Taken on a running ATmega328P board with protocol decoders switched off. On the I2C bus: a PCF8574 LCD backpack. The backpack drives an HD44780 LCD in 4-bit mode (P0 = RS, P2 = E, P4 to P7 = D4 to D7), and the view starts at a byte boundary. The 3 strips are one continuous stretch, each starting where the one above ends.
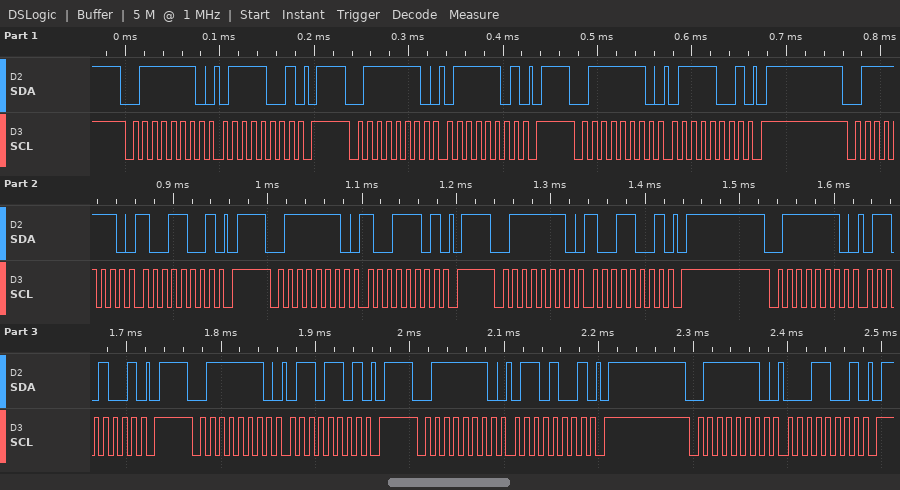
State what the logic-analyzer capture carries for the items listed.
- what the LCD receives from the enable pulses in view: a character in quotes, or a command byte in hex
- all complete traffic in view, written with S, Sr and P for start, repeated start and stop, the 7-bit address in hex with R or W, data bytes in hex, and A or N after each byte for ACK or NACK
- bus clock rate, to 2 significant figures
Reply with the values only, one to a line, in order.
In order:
'y'
S 3FW A 79 A P S 3FW A 7D A P S 3FW A 79 A P S 3FW A 99 A P S 3FW A 9D A P S 3FW A 99 A P S 3FW A 69 A P S 3FW A 6D A P S 3FW A 69 A P S 3FW A 19 A P
100 kHz
